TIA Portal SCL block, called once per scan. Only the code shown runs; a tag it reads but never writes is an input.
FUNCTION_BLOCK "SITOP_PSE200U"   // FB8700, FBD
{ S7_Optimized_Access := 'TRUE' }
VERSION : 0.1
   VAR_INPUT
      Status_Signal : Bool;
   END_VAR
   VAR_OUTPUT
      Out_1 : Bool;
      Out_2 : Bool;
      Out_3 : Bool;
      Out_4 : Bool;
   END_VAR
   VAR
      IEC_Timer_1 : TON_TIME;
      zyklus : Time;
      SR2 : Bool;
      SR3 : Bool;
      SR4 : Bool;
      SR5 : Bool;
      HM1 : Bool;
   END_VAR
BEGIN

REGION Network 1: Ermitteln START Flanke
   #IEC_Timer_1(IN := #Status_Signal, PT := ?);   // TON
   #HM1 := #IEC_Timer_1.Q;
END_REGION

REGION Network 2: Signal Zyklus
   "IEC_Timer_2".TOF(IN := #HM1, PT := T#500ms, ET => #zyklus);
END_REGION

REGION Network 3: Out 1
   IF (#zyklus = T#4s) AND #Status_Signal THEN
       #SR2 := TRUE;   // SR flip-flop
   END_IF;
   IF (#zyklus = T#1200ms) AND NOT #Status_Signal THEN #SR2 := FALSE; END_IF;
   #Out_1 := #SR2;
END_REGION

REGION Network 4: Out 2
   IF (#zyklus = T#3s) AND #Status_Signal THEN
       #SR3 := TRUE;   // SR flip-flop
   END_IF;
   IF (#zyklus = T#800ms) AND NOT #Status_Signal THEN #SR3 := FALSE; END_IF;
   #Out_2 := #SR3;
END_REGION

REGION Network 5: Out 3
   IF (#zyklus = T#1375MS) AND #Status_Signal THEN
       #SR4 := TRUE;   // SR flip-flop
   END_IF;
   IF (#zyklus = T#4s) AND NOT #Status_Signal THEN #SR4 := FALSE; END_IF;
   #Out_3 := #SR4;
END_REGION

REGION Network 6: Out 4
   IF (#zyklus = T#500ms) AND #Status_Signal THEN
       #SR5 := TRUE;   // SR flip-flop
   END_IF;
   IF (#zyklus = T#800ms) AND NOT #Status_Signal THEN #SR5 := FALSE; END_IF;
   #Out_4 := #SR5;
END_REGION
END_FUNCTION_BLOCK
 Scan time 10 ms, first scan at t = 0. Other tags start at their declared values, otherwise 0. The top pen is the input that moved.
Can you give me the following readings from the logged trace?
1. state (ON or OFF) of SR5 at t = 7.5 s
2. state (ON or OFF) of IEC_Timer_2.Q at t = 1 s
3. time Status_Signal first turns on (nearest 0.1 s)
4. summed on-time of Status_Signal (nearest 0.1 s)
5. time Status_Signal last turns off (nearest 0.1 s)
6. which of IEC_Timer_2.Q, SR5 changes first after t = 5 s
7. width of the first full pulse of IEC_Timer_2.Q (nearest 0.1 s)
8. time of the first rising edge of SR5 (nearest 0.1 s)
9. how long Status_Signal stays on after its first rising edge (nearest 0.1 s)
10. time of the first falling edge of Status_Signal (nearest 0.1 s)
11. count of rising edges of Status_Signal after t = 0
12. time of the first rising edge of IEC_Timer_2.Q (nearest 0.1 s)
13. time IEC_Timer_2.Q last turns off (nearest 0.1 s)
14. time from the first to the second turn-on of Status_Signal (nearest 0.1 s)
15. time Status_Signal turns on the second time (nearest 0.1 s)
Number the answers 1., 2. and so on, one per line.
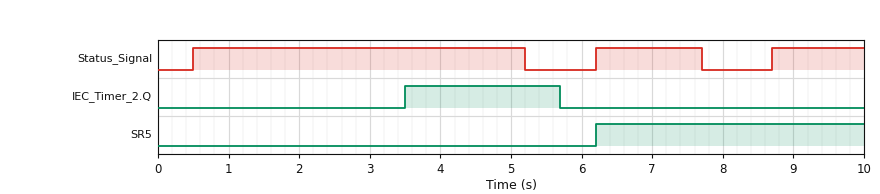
1. ON
2. OFF
3. 0.5 s
4. 7.5 s
5. 7.7 s
6. IEC_Timer_2.Q
7. 2.2 s
8. 6.2 s
9. 4.7 s
10. 5.2 s
11. 3
12. 3.5 s
13. 5.7 s
14. 5.7 s
15. 6.2 s
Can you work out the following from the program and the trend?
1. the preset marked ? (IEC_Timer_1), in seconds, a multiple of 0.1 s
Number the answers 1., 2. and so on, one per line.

1. 3.0 s
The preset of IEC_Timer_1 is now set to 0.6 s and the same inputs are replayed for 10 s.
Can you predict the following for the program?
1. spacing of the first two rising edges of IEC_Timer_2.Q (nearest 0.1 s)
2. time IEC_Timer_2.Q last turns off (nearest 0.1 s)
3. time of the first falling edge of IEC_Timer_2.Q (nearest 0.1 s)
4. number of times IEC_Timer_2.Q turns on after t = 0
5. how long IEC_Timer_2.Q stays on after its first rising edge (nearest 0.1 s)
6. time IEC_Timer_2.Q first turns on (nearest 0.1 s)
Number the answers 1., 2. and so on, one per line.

1. 5.7 s
2. 8.2 s
3. 5.7 s
4. 3
5. 4.6 s
6. 1.1 s
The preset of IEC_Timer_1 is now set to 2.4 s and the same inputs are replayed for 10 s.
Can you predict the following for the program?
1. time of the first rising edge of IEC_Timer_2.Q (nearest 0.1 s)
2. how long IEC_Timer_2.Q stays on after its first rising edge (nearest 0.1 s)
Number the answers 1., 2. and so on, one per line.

1. 2.9 s
2. 2.8 s
